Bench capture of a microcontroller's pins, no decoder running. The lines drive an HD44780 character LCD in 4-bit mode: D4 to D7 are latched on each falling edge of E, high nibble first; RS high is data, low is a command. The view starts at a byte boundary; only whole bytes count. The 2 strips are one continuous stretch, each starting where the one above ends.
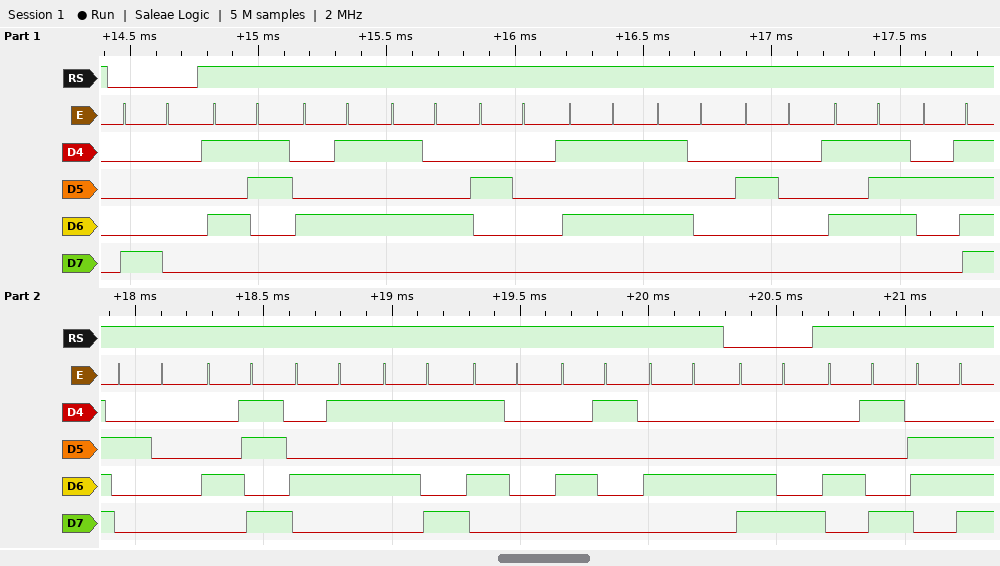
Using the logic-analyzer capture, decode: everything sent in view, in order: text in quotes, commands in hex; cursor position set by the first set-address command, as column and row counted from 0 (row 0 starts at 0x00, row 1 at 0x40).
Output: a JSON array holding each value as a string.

["0x80 \"SET UP W/ KEYPAD\" 0xC8 \"In\"", "column 0, row 0"]
